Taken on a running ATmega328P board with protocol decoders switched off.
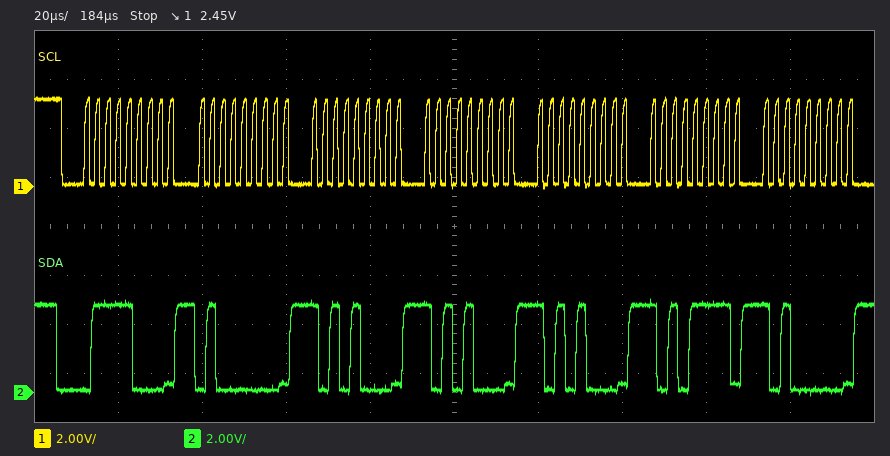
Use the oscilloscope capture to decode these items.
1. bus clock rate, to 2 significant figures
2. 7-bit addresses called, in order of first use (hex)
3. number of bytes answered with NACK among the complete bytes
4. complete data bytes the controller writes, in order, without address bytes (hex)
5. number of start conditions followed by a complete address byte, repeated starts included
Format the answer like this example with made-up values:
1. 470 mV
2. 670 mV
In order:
1. 400 kHz
2. 0x3C
3. 0
4. 40 A8 A8 A8 AF A0
5. 1
